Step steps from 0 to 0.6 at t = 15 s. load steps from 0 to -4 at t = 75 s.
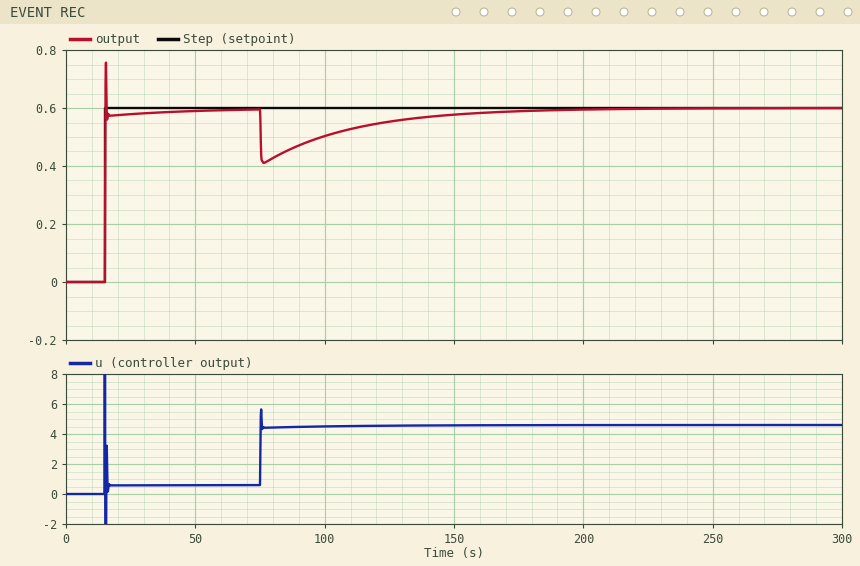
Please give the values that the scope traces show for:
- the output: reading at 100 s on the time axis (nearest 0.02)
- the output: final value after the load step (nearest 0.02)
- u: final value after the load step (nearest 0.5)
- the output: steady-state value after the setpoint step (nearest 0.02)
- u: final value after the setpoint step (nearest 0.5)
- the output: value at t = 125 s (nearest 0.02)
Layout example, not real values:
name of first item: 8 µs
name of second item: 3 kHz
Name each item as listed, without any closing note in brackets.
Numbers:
the output: reading at 100 s on the time axis: 0.50
the output: final value after the load step: 0.60
u: final value after the load step: 4.5
the output: steady-state value after the setpoint step: 0.60
u: final value after the setpoint step: 0.5
the output: value at t = 125 s: 0.56
